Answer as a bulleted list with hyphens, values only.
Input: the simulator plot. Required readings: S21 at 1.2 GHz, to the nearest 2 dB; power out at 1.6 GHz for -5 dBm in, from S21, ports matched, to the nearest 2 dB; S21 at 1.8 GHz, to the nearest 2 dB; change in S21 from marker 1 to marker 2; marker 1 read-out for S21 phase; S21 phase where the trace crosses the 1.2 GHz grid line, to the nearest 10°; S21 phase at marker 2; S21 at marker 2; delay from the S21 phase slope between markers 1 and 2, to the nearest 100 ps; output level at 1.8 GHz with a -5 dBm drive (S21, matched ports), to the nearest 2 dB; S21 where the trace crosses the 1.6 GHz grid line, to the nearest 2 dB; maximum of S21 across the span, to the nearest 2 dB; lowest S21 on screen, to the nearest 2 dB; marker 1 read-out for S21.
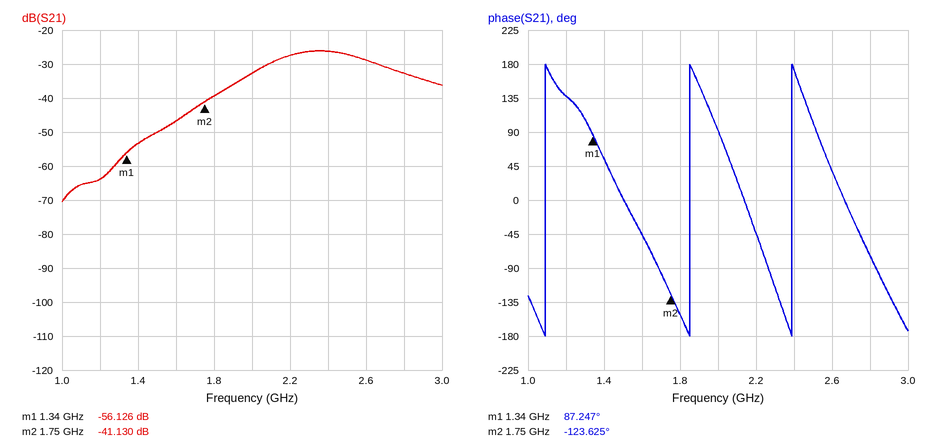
- -64 dB
- -52 dBm
- -40 dB
- 14.996 dB
- 87.247°
- 140°
- -123.625°
- -41.130 dB
- 1.4 ns
- -44 dBm
- -46 dB
- -26 dB
- -70 dB
- -56.126 dB
